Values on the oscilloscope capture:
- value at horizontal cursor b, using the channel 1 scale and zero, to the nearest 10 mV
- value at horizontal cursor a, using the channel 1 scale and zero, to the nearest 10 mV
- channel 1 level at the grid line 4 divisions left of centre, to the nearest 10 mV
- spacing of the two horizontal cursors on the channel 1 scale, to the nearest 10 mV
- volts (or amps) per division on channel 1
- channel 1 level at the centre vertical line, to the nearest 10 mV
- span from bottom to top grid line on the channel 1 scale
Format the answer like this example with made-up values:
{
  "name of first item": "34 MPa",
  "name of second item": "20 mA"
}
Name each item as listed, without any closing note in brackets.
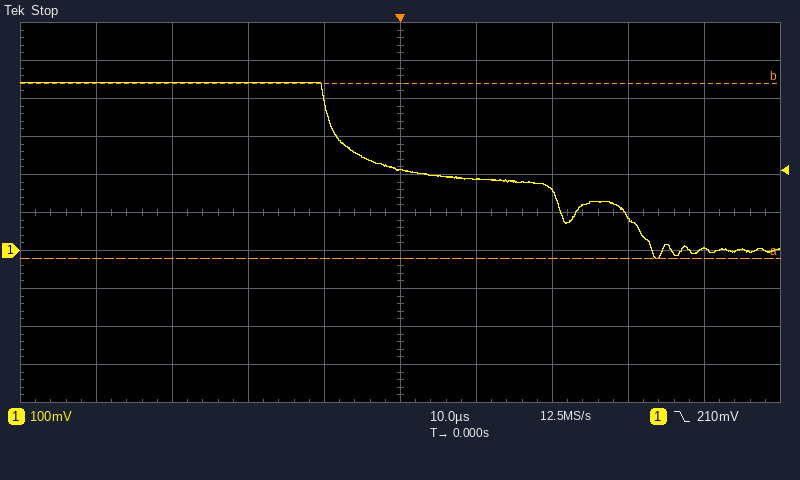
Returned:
{
  "value at horizontal cursor b, using the channel 1 scale and zero, to the nearest 10 mV": "440 mV",
  "value at horizontal cursor a, using the channel 1 scale and zero, to the nearest 10 mV": "-20 mV",
  "channel 1 level at the grid line 4 divisions left of centre, to the nearest 10 mV": "440 mV",
  "spacing of the two horizontal cursors on the channel 1 scale, to the nearest 10 mV": "460 mV",
  "volts (or amps) per division on channel 1": "100 mV",
  "channel 1 level at the centre vertical line, to the nearest 10 mV": "210 mV",
  "span from bottom to top grid line on the channel 1 scale": "1 V"
}
